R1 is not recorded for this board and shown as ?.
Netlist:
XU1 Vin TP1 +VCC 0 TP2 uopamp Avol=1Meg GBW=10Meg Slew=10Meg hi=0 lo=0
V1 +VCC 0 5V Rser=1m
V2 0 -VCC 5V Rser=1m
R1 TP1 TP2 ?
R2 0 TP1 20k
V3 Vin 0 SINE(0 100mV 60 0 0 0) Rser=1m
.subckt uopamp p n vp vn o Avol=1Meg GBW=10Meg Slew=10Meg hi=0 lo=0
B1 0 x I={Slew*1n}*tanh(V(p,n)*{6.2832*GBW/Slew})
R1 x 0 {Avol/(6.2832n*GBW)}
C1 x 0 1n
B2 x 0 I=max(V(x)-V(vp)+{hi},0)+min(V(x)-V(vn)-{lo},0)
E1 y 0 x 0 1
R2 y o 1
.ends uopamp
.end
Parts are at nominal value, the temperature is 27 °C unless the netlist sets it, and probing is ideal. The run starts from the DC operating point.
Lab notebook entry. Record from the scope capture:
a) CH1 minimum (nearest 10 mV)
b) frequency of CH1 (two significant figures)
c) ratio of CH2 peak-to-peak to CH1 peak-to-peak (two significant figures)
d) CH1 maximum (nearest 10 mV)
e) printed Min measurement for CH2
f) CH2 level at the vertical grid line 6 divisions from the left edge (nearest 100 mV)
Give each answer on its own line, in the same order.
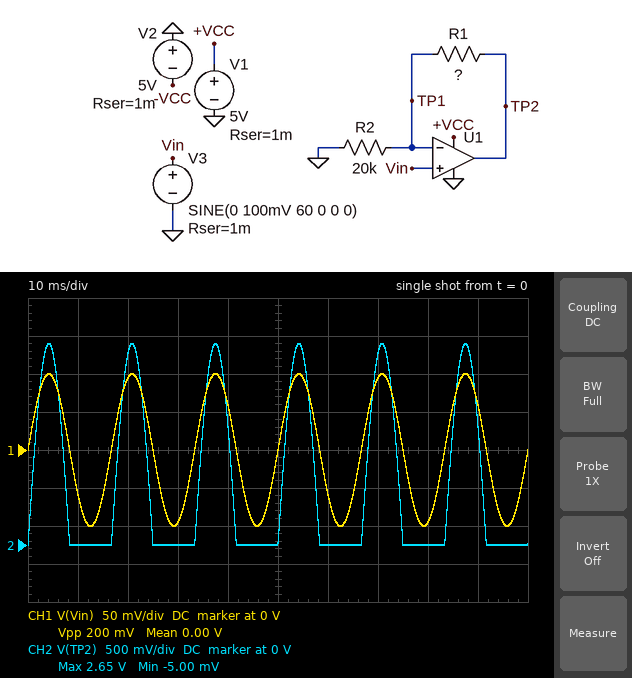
-100 mV
60 Hz
13
100 mV
-5.00 mV
0 V
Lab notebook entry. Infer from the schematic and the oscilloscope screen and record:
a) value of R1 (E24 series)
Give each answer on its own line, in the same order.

510 kΩ
